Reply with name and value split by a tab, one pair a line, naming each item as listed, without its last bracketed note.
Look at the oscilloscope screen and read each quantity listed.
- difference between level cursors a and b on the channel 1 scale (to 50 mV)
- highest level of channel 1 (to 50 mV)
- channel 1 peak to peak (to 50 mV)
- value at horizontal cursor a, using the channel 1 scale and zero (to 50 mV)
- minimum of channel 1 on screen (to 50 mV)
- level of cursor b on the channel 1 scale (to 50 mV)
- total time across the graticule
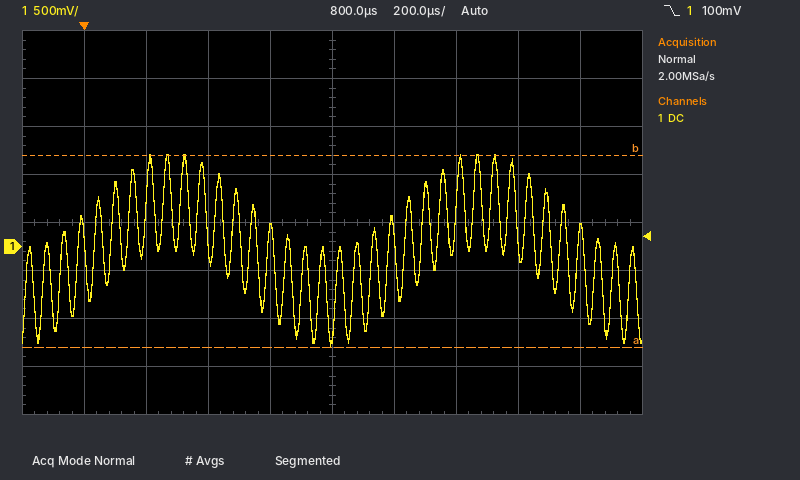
difference between level cursors a and b on the channel 1 scale	2.00 V
highest level of channel 1	950 mV
channel 1 peak to peak	2.00 V
value at horizontal cursor a, using the channel 1 scale and zero	-1.05 V
minimum of channel 1 on screen	-1.05 V
level of cursor b on the channel 1 scale	950 mV
total time across the graticule	2 ms
